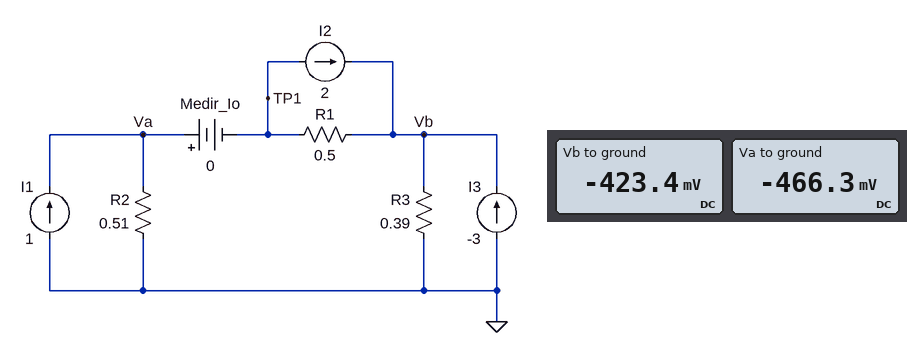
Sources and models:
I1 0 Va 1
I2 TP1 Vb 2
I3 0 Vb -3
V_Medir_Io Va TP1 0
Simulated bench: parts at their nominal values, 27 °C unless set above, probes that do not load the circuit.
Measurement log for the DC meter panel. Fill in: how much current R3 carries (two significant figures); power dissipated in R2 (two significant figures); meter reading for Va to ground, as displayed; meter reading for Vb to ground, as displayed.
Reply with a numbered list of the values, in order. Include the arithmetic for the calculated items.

1. (0 V - (-423.4 mV)) / 390 mΩ = 1.1 A
2. (0 V - (-466.3 mV))^2 / 510 mΩ = 430 mW
3. -466.3 mV
4. -423.4 mV
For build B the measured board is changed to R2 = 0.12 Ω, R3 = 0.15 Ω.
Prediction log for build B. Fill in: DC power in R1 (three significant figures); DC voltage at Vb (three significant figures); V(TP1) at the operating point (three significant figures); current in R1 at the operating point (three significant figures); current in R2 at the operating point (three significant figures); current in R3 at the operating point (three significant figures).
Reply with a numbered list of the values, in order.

1. 759 µW
2. -144 mV
3. -125 mV
4. 39.0 mA
5. 1.04 A
6. 961 mA
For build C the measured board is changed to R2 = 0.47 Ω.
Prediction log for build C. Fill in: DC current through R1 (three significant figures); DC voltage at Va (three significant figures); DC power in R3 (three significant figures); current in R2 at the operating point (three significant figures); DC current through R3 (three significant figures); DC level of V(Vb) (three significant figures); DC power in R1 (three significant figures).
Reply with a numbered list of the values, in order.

1. 58.8 mA
2. -442 mV
3. 437 mW
4. 941 mA
5. 1.06 A
6. -413 mV
7. 1.73 mW
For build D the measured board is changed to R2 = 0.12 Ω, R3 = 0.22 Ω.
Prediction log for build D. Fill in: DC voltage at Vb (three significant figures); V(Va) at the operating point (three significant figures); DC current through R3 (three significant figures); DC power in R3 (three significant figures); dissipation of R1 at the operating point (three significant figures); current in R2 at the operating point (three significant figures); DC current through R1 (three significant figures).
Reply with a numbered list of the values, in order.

1. -194 mV
2. -134 mV
3. 881 mA
4. 171 mW
5. 7.09 mW
6. 1.12 A
7. 119 mA
